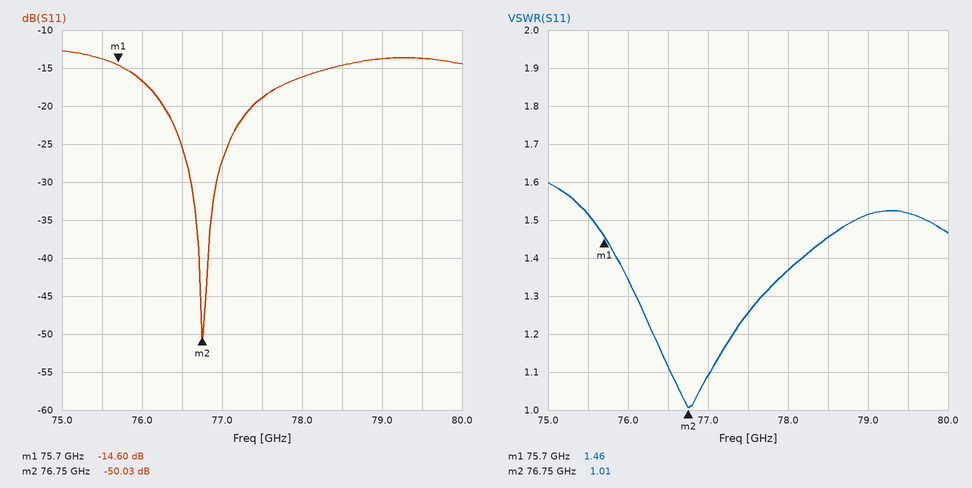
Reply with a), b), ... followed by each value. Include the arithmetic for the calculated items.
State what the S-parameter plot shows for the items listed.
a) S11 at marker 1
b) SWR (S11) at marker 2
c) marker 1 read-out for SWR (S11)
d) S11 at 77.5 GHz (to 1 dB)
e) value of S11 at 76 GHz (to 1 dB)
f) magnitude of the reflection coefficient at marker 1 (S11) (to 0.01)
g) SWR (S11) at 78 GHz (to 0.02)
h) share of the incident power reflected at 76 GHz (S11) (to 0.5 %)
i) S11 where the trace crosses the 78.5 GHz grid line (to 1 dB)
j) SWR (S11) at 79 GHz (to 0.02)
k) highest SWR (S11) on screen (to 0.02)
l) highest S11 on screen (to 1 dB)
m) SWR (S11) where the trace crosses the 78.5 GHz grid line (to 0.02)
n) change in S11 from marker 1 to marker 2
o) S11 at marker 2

a) -14.60 dB
b) 1.01
c) 1.46
d) -19 dB
e) -17 dB
f) 10^(-14.6/20) ≈ 0.19
g) 1.36
h) 10^(-17/10) ≈ 2.0 %
i) -15 dB
j) 1.52
k) 1.60
l) -13 dB
m) 1.46
n) -50.03 − (-14.6) = -35.43 dB
o) -50.03 dB
